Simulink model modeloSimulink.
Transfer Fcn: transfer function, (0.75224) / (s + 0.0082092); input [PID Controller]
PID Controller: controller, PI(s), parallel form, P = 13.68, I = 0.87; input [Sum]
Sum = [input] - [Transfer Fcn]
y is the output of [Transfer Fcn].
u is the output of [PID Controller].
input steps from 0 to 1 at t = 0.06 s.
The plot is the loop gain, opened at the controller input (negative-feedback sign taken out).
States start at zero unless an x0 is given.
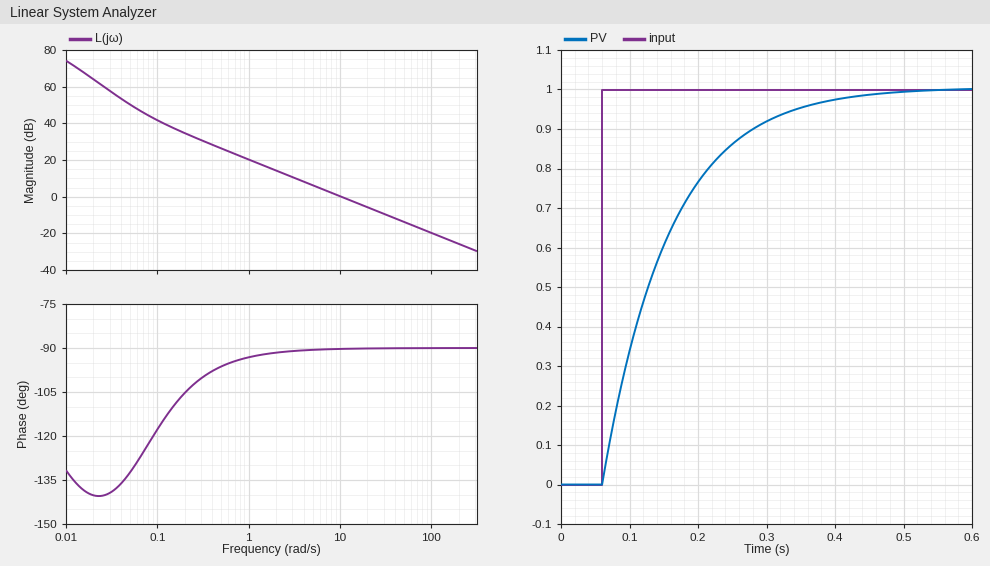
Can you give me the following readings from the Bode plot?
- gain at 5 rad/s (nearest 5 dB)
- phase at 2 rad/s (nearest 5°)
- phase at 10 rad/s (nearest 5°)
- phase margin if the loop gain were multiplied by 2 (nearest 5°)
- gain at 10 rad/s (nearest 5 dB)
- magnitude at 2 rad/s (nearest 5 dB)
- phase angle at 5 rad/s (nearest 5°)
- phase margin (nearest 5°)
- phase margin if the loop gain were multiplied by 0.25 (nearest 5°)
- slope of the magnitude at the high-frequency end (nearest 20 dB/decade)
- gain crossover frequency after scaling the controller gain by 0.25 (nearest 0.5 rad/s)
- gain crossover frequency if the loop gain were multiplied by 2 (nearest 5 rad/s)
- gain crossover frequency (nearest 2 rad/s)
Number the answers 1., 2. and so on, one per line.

1. 5 dB
2. -90°
3. -90°
4. 90°
5. 0 dB
6. 15 dB
7. -90°
8. 90°
9. 90°
10. -20 dB/decade
11. 2.5 rad/s
12. 20 rad/s
13. 10 rad/s
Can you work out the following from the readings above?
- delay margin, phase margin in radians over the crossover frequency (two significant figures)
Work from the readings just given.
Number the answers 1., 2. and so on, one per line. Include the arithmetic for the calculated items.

1. 90 × π / 180 / 10 = 0.16 s
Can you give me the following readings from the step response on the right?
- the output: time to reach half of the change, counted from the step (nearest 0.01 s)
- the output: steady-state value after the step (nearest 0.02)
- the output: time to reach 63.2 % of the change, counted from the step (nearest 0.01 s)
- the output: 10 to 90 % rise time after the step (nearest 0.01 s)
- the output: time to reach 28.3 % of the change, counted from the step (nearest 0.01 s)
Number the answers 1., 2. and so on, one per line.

1. 0.07 s
2. 1.00
3. 0.10 s
4. 0.21 s
5. 0.03 s
